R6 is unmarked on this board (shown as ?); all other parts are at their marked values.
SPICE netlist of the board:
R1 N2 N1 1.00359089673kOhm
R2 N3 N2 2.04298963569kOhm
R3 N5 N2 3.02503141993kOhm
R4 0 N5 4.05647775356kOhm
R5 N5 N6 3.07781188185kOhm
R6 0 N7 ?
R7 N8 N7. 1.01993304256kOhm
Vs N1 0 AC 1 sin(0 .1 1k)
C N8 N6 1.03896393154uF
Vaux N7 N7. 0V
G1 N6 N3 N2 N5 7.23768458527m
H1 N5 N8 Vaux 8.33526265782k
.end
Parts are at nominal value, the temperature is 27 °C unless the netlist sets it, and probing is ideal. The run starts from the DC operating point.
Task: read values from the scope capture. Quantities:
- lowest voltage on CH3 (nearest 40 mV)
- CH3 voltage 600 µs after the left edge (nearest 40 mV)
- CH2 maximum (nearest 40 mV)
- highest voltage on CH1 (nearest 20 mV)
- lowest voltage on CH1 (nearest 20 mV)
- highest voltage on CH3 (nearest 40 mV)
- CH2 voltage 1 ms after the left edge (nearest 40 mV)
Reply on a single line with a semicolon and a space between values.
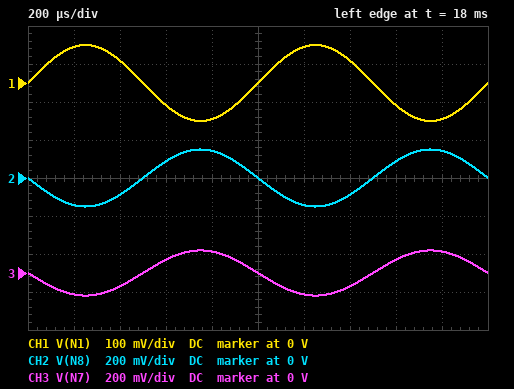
-120 mV; 80 mV; 160 mV; 100 mV; -100 mV; 120 mV; 0 V
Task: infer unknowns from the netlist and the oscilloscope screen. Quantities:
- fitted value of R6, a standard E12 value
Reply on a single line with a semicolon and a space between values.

3.9 kΩ
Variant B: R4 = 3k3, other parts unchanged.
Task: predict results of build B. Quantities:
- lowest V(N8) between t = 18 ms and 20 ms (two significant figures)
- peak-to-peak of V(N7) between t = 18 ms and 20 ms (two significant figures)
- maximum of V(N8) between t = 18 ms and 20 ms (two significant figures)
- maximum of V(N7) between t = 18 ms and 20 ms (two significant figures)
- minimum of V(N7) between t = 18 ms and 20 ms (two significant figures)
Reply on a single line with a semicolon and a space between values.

-140 mV; 230 mV; 140 mV; 110 mV; -110 mV
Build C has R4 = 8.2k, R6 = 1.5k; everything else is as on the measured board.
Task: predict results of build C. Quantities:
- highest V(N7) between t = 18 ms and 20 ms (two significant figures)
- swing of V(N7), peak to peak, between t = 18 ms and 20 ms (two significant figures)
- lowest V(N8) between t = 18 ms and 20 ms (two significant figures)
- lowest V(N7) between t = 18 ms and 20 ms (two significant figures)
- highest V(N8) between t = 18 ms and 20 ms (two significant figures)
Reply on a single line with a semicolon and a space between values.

27 mV; 54 mV; -45 mV; -27 mV; 45 mV
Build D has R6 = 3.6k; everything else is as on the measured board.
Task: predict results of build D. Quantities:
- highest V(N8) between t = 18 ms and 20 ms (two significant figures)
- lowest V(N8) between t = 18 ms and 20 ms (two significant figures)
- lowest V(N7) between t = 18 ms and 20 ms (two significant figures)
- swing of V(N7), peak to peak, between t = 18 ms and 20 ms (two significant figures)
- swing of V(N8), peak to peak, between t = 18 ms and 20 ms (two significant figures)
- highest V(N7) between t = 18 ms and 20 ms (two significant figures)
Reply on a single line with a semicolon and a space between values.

130 mV; -130 mV; -99 mV; 200 mV; 250 mV; 99 mV
